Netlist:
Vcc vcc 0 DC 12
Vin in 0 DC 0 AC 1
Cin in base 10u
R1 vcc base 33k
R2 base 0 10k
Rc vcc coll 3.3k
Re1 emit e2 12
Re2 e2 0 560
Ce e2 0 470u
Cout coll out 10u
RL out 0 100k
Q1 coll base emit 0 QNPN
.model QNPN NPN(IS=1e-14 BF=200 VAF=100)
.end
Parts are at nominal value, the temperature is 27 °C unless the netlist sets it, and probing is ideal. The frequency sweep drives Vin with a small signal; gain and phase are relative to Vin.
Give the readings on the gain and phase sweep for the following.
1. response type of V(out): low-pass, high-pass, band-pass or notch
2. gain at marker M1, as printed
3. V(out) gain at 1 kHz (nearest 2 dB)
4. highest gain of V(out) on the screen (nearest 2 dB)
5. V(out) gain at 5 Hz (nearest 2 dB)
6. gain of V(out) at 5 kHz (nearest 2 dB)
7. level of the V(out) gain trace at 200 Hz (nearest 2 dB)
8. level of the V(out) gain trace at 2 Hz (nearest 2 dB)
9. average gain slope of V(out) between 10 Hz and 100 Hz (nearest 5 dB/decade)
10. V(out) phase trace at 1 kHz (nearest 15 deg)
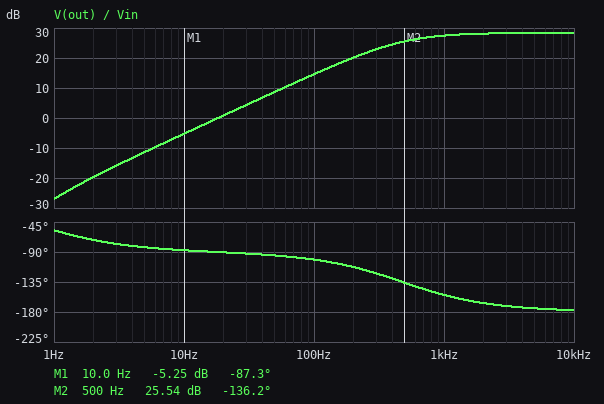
high-pass
-5.25 dB
28 dB
28 dB
-12 dB
28 dB
20 dB
-20 dB
20 dB/decade
-150 deg
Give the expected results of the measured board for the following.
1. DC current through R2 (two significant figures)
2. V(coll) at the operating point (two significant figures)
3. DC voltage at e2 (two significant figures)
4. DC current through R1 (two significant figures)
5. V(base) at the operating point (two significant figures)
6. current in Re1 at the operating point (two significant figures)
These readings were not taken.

250 µA
1.9 V
1.7 V
290 µA
2.5 V
3.1 mA
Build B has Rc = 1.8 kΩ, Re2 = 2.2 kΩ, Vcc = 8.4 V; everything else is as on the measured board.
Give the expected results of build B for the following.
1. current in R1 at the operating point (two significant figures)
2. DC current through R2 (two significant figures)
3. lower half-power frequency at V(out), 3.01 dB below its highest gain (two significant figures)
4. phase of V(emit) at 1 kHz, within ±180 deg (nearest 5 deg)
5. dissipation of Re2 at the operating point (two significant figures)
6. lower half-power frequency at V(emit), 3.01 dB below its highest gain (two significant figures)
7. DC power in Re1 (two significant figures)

200 µA
190 µA
8.2 Hz
0 deg
750 µW
1.2 Hz
4.1 µW
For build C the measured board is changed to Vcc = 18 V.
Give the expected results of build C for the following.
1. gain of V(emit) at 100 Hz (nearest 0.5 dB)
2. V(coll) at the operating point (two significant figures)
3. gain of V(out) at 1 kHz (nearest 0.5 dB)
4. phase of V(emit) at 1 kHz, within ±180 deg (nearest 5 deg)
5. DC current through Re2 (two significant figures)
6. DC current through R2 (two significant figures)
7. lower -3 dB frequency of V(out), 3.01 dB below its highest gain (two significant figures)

-21.5 dB
2.8 V
20.0 dB
30 deg
4.7 mA
340 µA
670 Hz
